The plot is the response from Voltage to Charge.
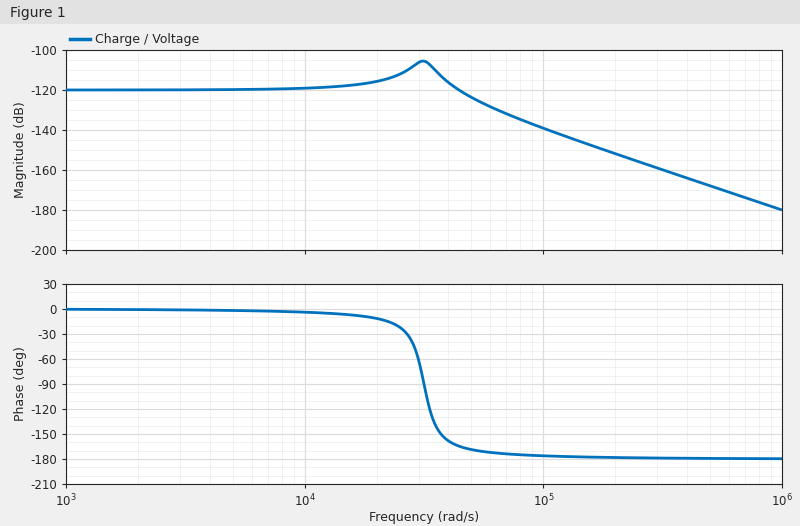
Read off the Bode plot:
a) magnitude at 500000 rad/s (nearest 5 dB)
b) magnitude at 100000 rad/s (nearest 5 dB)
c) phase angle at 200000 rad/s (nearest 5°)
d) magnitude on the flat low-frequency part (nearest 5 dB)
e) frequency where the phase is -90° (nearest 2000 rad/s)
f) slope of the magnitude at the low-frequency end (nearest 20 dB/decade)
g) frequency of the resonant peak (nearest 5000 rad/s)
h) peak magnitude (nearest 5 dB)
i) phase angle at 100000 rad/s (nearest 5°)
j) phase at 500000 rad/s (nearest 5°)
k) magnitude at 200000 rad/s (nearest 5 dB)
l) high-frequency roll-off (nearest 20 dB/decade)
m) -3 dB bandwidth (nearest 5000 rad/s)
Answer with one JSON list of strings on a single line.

["-170 dB", "-140 dB", "-180°", "-120 dB", "32000 rad/s", "0 dB/decade", "30000 rad/s", "-105 dB", "-175°", "-180°", "-150 dB", "-40 dB/decade", "50000 rad/s"]
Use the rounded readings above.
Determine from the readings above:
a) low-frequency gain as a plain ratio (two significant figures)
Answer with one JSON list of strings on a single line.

["0.0000010"]
